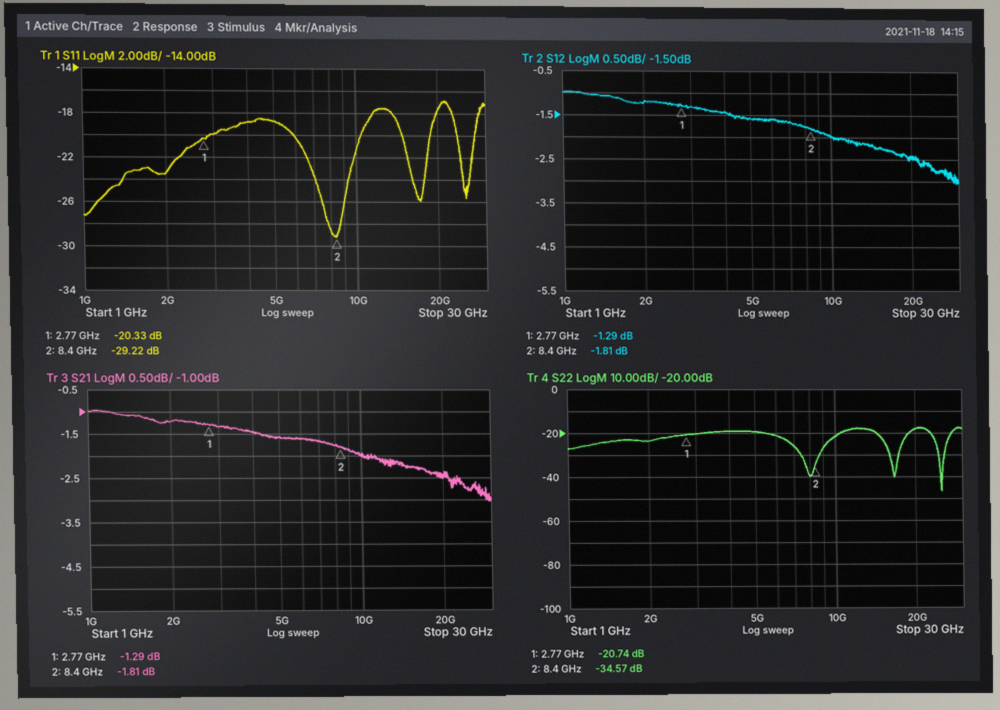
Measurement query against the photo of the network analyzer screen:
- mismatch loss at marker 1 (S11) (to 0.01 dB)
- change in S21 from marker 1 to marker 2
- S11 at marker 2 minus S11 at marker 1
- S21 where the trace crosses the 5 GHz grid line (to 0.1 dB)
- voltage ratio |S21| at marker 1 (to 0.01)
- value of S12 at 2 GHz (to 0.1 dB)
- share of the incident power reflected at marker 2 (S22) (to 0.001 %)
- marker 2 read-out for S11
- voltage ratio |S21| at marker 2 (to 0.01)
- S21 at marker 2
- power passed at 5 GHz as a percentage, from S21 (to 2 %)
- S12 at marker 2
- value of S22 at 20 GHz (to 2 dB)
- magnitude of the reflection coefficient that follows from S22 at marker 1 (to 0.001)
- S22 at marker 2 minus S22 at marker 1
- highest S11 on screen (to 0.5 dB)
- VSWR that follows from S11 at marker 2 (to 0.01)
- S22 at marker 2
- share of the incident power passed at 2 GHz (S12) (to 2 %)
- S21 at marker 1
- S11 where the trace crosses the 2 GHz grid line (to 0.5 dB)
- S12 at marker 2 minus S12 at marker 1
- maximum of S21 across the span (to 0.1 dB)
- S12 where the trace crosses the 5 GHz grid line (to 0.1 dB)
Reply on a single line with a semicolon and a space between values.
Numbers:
0.04 dB; -0.52 dB; -8.89 dB; -1.6 dB; 0.86; -1.2 dB; 0.035 %; -29.22 dB; 0.81; -1.81 dB; 70 %; -1.81 dB; -18 dB; 0.092; -13.83 dB; -17.0 dB; 1.07; -34.57 dB; 76 %; -1.29 dB; -23.5 dB; -0.52 dB; -1.0 dB; -1.6 dB
